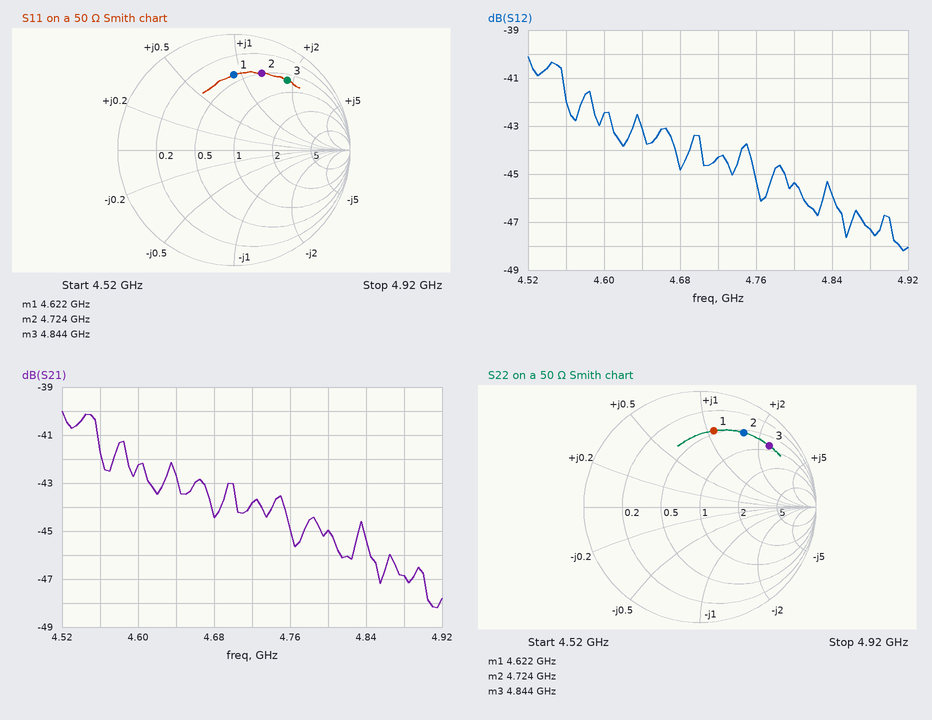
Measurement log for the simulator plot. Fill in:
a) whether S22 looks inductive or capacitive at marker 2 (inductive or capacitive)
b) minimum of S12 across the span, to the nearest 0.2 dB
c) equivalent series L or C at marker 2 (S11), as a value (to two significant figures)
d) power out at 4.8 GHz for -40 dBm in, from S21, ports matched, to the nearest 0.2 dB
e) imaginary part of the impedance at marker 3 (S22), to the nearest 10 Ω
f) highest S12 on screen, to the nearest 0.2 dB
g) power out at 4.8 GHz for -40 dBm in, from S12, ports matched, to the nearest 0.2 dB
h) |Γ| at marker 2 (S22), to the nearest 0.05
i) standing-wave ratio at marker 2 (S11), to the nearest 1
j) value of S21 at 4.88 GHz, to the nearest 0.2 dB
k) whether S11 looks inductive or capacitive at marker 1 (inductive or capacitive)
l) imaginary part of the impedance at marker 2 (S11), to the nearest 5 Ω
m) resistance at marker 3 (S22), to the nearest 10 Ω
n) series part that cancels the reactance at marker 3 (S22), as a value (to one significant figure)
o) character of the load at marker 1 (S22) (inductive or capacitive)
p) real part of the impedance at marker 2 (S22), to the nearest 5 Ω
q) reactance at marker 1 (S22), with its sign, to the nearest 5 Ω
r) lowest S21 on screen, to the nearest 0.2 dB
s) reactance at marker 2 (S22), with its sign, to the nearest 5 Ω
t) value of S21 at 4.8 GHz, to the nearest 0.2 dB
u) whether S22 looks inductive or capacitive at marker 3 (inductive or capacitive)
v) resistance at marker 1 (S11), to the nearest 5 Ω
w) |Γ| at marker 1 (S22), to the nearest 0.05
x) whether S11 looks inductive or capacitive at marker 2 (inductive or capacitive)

inductive
-48.2 dB
2.2 nH
-85.0 dBm
+120 Ω
-40.2 dB
-85.4 dBm
0.75
6
-46.8 dB
inductive
+65 Ω
40 Ω
300 fF
inductive
30 Ω
+55 Ω
-48.2 dB
+80 Ω
-45.0 dB
inductive
20 Ω
0.65
inductive
